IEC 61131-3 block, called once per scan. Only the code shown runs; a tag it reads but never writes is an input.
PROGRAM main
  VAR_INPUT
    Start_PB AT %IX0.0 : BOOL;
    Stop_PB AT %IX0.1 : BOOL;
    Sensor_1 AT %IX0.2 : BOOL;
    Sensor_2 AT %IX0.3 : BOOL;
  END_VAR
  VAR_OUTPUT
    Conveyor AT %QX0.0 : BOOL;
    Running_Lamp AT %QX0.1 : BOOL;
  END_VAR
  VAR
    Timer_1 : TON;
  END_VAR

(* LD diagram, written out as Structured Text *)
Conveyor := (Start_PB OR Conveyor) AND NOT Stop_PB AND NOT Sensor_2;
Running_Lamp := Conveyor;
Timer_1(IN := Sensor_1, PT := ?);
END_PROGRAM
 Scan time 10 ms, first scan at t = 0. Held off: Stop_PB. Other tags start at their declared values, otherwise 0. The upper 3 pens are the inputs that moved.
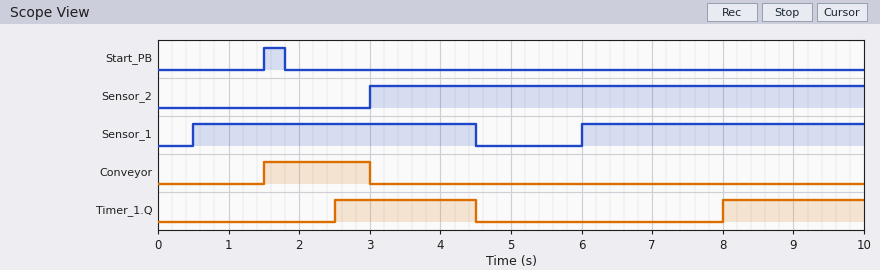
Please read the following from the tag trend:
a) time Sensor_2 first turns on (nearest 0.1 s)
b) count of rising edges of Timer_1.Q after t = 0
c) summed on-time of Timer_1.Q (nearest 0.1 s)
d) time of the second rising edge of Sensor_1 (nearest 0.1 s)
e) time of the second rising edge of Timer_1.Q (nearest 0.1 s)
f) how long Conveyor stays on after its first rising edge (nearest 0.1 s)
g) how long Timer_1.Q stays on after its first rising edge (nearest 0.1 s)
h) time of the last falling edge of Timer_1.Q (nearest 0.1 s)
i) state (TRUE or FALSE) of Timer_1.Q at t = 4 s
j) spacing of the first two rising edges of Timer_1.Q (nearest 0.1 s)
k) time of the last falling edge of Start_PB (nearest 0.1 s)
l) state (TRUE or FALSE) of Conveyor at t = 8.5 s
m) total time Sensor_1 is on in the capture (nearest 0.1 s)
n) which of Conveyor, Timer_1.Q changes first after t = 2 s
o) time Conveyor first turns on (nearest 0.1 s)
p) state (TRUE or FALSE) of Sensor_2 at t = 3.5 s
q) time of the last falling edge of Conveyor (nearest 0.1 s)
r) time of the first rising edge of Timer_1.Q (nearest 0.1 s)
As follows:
3.0 s
2
4.0 s
6.0 s
8.0 s
1.5 s
2.0 s
4.5 s
TRUE
5.5 s
1.8 s
FALSE
8.0 s
Timer_1.Q
1.5 s
TRUE
3.0 s
2.5 s
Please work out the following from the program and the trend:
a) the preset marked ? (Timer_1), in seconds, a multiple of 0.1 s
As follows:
2.0 s
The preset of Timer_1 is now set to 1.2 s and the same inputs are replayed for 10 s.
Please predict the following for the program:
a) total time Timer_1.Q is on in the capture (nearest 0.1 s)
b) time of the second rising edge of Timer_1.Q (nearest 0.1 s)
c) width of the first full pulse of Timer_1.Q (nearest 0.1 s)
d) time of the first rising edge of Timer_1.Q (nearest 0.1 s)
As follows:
5.6 s
7.2 s
2.8 s
1.7 s
